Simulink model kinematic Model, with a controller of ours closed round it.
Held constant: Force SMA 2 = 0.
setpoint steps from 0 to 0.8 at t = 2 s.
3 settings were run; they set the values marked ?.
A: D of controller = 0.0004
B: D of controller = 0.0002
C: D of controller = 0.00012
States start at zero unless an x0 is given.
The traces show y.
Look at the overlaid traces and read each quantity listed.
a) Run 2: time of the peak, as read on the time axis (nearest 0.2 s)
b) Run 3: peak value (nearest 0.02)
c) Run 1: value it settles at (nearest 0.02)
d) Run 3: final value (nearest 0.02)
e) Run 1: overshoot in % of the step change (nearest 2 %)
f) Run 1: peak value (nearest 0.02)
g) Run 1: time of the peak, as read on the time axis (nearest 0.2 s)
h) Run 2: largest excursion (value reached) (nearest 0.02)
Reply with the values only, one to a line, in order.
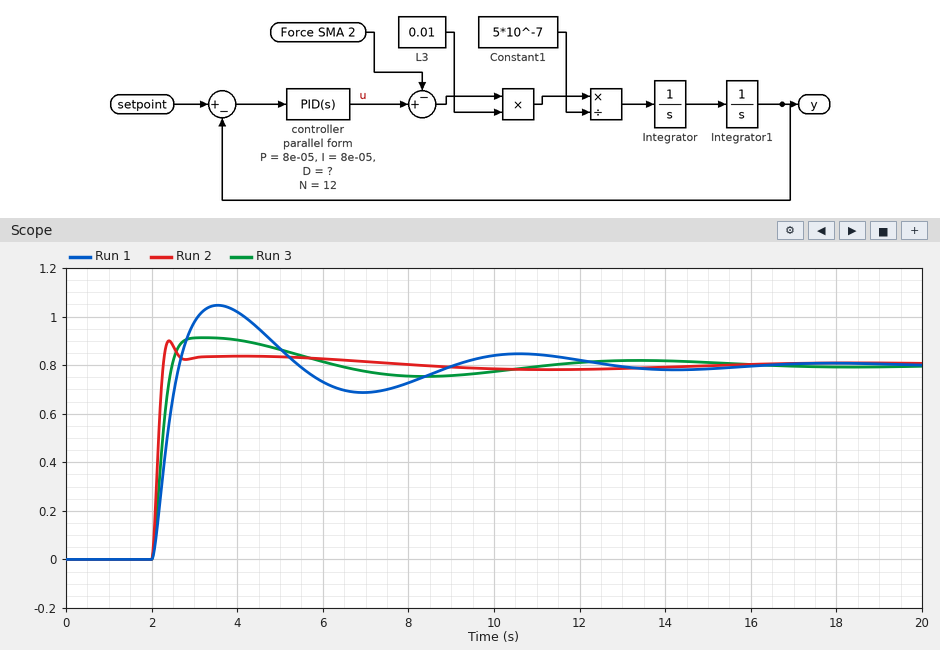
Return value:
2.4 s
0.92
0.80
0.80
30 %
1.04
3.6 s
0.90
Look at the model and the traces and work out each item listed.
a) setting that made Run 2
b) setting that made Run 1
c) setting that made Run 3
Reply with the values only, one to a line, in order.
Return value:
A
C
B
